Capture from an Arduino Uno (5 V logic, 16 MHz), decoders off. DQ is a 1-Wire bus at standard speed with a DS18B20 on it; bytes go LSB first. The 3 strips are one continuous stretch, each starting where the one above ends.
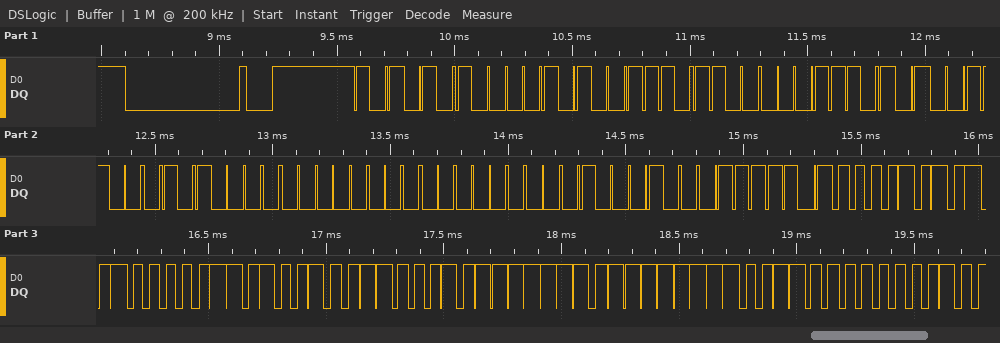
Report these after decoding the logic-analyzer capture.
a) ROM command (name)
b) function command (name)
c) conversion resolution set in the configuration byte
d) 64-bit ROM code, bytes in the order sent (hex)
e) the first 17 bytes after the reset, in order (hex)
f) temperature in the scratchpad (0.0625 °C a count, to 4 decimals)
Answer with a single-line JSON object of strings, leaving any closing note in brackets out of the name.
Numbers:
{"ROM command": "Match ROM", "function command": "Read Scratchpad", "conversion resolution set in the configuration byte": "12 bits", "64-bit ROM code, bytes in the order sent": "28 37 B8 32 0A 00 00 22", "the first 17 bytes after the reset, in order": "55 28 37 B8 32 0A 00 00 22 BE 50 05 4B 46 7F FF 0C", "temperature in the scratchpad": "85.0000 °C"}
